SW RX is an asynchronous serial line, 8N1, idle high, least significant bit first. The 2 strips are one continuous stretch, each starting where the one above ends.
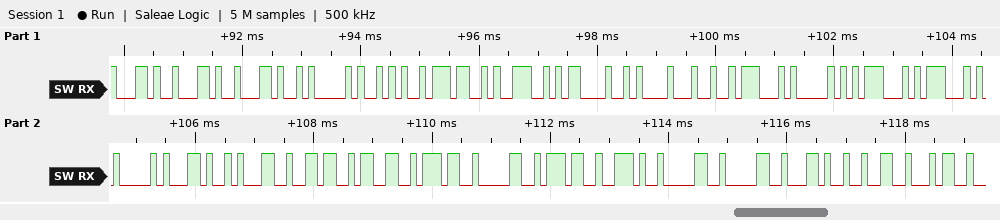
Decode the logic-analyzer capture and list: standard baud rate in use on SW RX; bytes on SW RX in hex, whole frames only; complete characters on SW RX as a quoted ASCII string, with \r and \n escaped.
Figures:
9600 baud
2C 2C 2C 41 2A 37 39 0D 0A 24 47 50 47 47 41 2C 31 36 33 37 30 37 2E 30 30 2C 32 34
",,,A*79\r\n$GPGGA,163707.00,24"
